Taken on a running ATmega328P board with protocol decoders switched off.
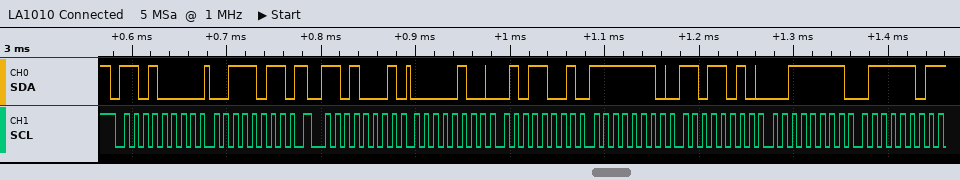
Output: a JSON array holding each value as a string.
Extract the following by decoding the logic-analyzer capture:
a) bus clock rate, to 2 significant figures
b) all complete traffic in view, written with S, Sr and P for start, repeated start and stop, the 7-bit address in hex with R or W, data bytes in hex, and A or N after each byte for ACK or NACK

["100 kHz", "S 68W A 3B A Sr 68R A 04 A 59 A FE A DA A 3F A 7D N"]
